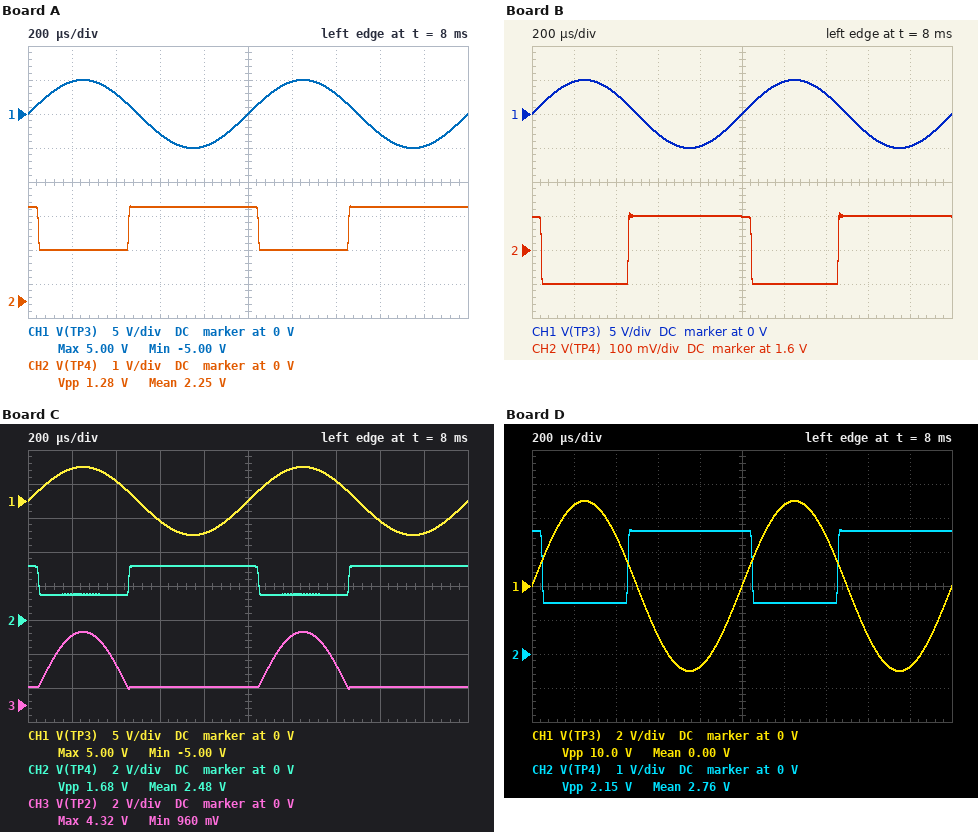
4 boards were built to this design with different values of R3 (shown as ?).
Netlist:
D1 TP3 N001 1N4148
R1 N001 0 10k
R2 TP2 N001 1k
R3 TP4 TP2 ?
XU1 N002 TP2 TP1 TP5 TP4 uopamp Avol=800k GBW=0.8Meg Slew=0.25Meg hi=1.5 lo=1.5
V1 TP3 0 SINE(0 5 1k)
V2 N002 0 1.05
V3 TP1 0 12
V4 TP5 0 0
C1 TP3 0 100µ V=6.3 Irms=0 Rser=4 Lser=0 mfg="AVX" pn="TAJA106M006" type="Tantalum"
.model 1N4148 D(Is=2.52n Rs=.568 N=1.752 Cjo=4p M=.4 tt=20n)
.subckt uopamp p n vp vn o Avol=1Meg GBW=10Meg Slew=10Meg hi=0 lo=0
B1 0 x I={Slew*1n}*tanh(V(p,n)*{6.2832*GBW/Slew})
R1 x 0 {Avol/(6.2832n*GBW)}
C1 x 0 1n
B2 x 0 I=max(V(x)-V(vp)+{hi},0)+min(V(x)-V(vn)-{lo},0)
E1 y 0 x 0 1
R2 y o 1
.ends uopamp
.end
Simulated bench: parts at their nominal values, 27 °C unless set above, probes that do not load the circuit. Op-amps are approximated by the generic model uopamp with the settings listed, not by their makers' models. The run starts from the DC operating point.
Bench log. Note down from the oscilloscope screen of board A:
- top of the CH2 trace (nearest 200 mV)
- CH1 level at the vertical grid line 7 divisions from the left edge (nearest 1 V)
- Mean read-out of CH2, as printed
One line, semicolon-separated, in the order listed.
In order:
2.8 V; 3 V; 2.25 V
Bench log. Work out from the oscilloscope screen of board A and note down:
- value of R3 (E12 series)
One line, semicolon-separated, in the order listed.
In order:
18 kΩ
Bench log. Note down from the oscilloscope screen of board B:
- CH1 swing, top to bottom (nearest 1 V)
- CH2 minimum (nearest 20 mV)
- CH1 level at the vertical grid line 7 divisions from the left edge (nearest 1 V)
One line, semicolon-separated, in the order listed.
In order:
10 V; 1.50 V; 3 V
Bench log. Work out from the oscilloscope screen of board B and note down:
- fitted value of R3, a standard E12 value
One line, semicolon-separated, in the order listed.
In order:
6.8 kΩ
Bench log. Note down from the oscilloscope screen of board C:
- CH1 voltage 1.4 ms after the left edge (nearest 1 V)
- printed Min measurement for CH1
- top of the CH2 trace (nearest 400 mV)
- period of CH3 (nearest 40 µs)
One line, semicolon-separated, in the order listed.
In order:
3 V; -5.00 V; 3.2 V; 1.00 ms
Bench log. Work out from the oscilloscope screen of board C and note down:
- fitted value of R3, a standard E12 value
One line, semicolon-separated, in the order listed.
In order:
22 kΩ
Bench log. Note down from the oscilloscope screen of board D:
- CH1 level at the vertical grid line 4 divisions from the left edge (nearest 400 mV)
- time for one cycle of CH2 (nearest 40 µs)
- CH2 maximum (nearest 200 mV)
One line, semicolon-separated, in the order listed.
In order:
-4.8 V; 1.00 ms; 3.6 V
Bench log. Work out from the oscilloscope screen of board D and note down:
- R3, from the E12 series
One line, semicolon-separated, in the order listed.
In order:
27 kΩ
